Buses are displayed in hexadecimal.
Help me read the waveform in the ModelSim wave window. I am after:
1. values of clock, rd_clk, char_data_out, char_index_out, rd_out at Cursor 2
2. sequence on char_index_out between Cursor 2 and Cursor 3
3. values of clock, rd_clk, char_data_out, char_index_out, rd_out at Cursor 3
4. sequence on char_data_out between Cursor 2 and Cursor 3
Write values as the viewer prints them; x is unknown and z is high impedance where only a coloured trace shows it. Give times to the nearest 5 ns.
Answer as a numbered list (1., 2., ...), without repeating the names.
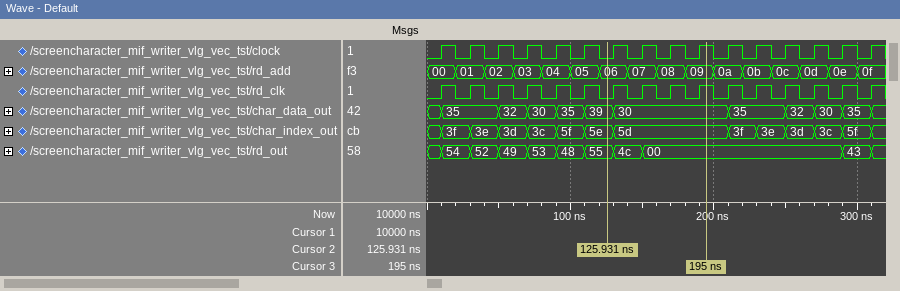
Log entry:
1. clock=0, rd_clk=0, char_data_out=39, char_index_out=5e, rd_out=55
2. 5e, 5d
3. clock=1, rd_clk=1, char_data_out=30, char_index_out=5d, rd_out=00
4. 39, 30
